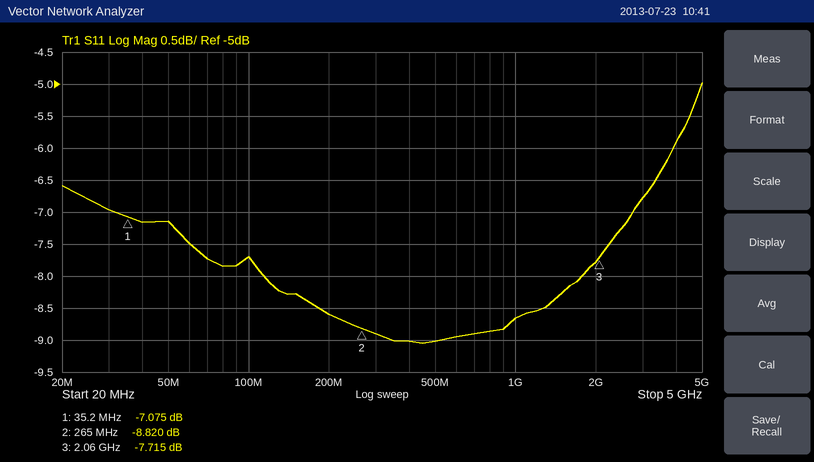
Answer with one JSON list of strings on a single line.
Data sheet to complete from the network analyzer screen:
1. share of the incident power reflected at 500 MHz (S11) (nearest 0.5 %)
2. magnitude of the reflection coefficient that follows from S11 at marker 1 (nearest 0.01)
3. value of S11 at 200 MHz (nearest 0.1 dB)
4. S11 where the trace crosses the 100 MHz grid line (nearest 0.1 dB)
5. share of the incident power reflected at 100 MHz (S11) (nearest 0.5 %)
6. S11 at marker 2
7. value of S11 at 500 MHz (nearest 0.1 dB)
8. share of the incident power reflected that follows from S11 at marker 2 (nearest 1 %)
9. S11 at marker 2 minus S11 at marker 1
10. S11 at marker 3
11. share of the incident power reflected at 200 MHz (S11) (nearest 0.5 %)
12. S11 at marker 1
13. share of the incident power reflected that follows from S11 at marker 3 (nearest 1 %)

["12.5 %", "0.44", "-8.6 dB", "-7.7 dB", "17.0 %", "-8.820 dB", "-9.0 dB", "13 %", "-1.745 dB", "-7.715 dB", "14.0 %", "-7.075 dB", "17 %"]
